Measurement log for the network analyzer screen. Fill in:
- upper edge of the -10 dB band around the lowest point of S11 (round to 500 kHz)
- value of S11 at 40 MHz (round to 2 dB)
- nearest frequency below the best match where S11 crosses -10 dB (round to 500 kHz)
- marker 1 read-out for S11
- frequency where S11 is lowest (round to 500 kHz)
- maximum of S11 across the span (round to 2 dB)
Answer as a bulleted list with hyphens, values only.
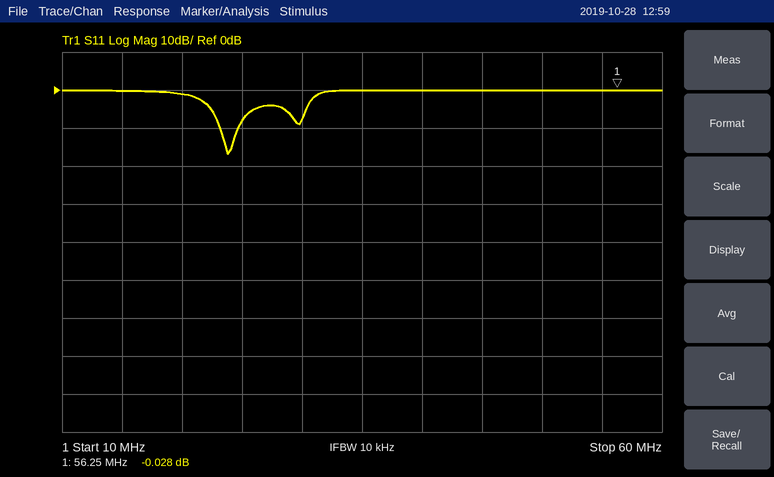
- 24.5 MHz
- 0 dB
- 23.0 MHz
- -0.028 dB
- 24.0 MHz
- 0 dB
